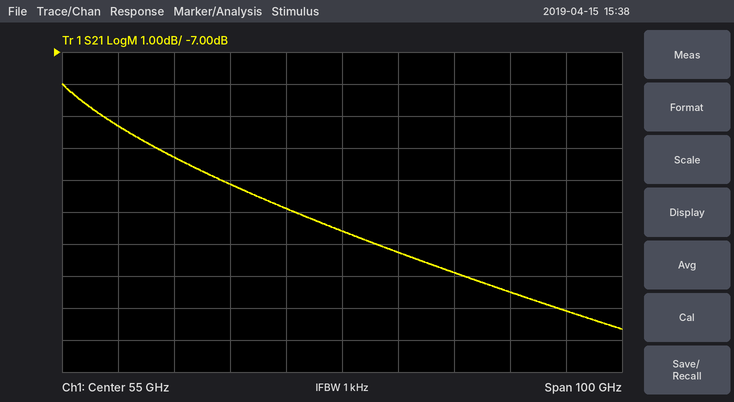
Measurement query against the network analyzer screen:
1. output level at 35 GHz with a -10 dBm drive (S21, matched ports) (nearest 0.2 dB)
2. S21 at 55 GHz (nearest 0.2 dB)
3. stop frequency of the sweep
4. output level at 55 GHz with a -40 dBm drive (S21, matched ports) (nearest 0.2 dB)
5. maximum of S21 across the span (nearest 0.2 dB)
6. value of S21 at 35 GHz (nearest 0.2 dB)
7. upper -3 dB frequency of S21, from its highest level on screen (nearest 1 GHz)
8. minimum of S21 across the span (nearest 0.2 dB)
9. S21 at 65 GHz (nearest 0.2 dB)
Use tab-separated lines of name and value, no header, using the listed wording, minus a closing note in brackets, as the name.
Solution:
output level at 35 GHz with a -10 dBm drive (S21, matched ports)	-21.2 dBm
S21 at 55 GHz	-12.6 dB
stop frequency of the sweep	105 GHz
output level at 55 GHz with a -40 dBm drive (S21, matched ports)	-52.6 dBm
maximum of S21 across the span	-8.0 dB
value of S21 at 35 GHz	-11.2 dB
upper -3 dB frequency of S21, from its highest level on screen	33 GHz
minimum of S21 across the span	-15.6 dB
S21 at 65 GHz	-13.2 dB
